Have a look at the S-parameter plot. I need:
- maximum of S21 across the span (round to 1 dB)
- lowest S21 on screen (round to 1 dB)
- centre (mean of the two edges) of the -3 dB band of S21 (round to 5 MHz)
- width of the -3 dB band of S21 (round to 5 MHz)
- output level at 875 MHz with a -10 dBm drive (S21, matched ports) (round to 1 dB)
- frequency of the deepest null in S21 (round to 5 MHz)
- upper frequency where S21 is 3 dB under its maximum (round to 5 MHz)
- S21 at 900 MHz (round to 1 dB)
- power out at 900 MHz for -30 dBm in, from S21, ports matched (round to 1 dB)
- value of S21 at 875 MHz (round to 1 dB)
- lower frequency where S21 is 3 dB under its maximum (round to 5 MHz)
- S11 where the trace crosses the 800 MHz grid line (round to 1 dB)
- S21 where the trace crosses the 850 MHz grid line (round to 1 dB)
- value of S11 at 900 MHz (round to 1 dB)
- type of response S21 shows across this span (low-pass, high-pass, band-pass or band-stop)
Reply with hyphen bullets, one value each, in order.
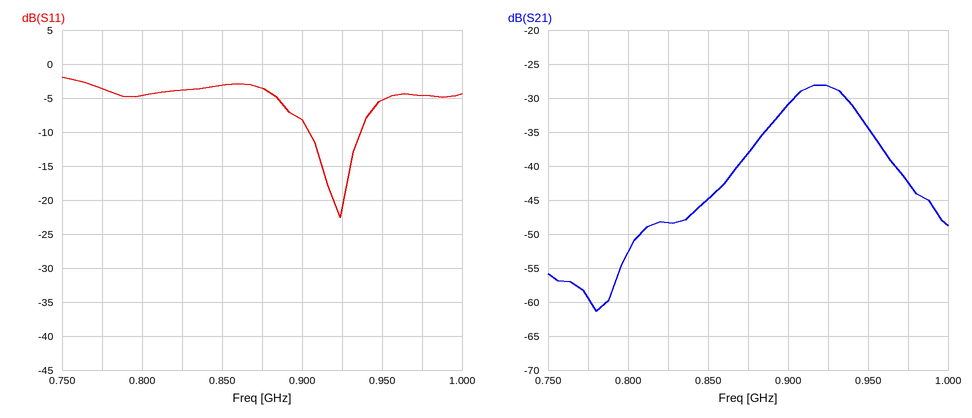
- -28 dB
- -61 dB
- 920 MHz
- 40 MHz
- -48 dBm
- 780 MHz
- 940 MHz
- -31 dB
- -61 dBm
- -38 dB
- 900 MHz
- -5 dB
- -45 dB
- -8 dB
- band-pass
